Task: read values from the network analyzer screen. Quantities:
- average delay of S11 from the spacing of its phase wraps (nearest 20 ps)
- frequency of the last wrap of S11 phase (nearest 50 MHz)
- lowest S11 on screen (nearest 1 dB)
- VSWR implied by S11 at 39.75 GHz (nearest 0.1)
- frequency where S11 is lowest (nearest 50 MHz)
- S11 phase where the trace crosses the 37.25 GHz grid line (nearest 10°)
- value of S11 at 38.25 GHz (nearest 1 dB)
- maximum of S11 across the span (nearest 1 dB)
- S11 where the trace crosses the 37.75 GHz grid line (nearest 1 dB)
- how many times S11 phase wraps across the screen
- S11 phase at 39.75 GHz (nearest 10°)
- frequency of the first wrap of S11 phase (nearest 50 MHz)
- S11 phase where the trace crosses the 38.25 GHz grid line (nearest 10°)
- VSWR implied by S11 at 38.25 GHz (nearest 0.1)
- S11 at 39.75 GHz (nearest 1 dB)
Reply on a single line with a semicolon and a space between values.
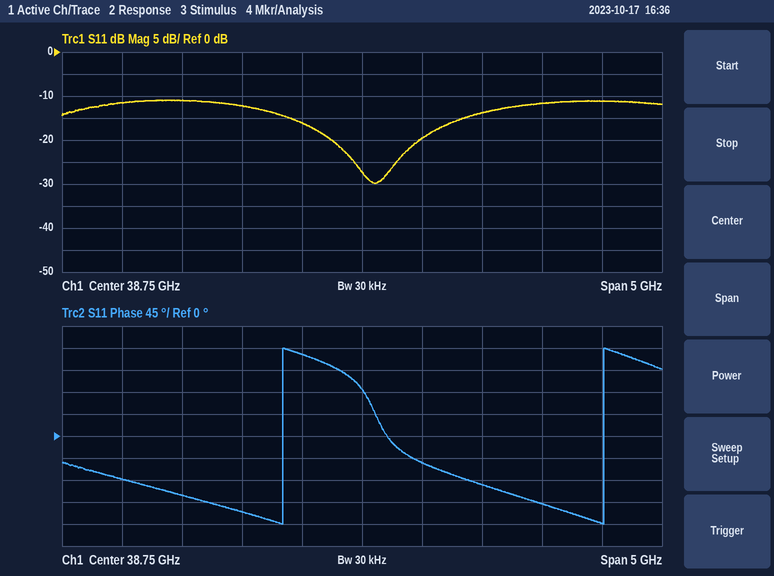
380 ps; 40.75 GHz; -30 dB; 1.5; 38.85 GHz; -120°; -16 dB; -11 dB; -12 dB; 2; -100°; 38.10 GHz; 170°; 1.4; -14 dB
